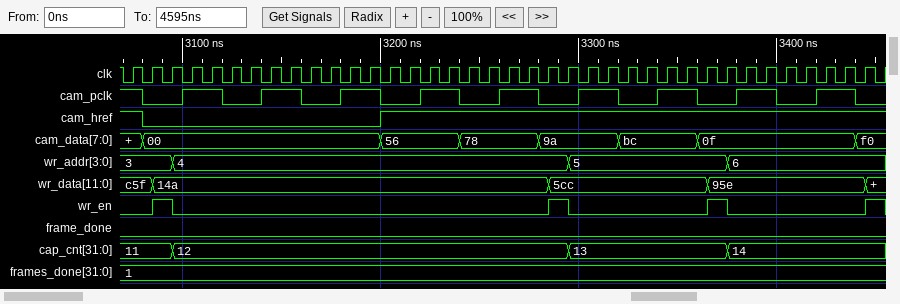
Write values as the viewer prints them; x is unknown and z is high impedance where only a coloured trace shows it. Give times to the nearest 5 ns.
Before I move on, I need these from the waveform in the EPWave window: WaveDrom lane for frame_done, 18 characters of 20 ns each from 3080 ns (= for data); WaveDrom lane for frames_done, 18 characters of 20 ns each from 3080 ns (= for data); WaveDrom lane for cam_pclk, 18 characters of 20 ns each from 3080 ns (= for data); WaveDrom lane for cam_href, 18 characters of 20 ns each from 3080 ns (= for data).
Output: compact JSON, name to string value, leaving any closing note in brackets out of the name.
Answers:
{"WaveDrom lane for frame_done, 18 characters of 20 ns each from 3080 ns": "{name: 'frame_done', wave: '0.................'}", "WaveDrom lane for frames_done, 18 characters of 20 ns each from 3080 ns": "{name: 'frames_done', wave: '=.................', data: '1'}", "WaveDrom lane for cam_pclk, 18 characters of 20 ns each from 3080 ns": "{name: 'cam_pclk', wave: '010101010101010101'}", "WaveDrom lane for cam_href, 18 characters of 20 ns each from 3080 ns": "{name: 'cam_href', wave: '0.....1...........'}"}
